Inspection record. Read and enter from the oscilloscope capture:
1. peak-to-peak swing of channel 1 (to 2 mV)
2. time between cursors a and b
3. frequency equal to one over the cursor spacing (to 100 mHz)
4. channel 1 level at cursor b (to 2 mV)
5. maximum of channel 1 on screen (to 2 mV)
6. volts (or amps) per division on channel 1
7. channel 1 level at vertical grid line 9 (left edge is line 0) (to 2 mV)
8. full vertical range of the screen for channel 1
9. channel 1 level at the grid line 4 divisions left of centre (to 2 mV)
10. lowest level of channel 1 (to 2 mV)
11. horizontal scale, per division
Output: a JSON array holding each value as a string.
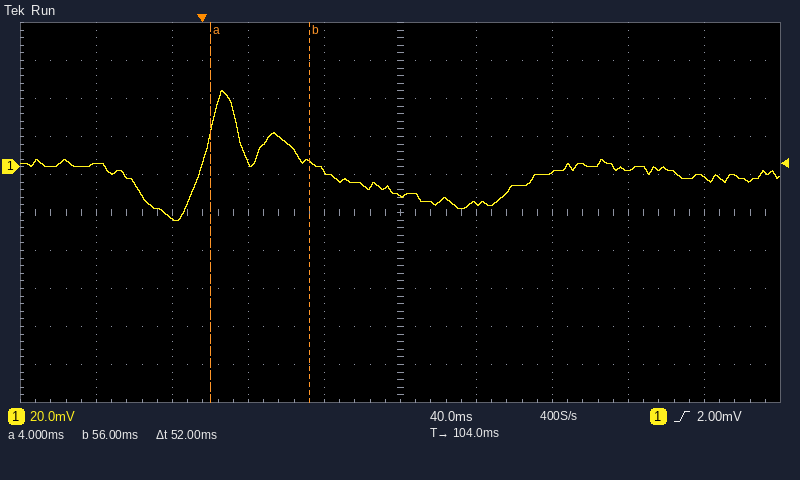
["68 mV", "52 ms", "19.2 Hz", "2 mV", "40 mV", "20 mV", "-6 mV", "200 mV", "2 mV", "-28 mV", "40 ms"]
